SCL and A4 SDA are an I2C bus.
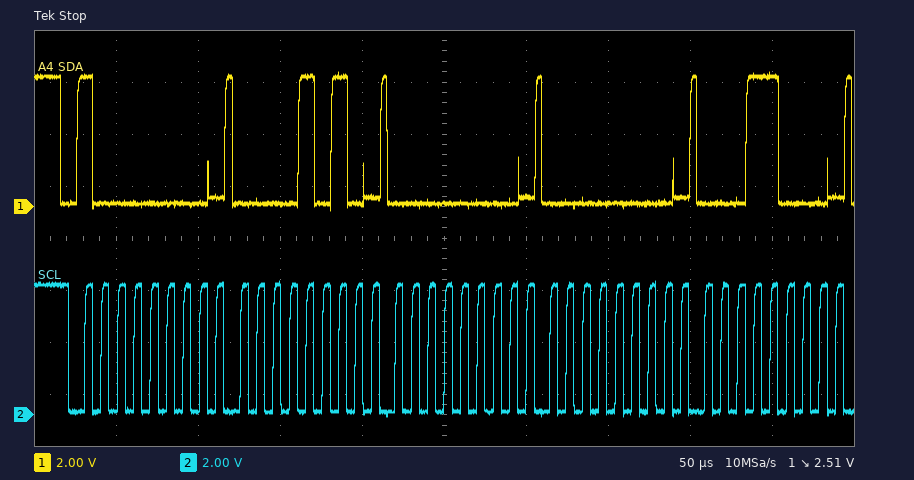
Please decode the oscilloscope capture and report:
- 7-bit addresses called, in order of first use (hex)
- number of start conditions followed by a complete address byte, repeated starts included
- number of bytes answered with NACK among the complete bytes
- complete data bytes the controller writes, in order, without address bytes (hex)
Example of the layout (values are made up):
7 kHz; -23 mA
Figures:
0x40; 1; 0; 0A 00 00 18
